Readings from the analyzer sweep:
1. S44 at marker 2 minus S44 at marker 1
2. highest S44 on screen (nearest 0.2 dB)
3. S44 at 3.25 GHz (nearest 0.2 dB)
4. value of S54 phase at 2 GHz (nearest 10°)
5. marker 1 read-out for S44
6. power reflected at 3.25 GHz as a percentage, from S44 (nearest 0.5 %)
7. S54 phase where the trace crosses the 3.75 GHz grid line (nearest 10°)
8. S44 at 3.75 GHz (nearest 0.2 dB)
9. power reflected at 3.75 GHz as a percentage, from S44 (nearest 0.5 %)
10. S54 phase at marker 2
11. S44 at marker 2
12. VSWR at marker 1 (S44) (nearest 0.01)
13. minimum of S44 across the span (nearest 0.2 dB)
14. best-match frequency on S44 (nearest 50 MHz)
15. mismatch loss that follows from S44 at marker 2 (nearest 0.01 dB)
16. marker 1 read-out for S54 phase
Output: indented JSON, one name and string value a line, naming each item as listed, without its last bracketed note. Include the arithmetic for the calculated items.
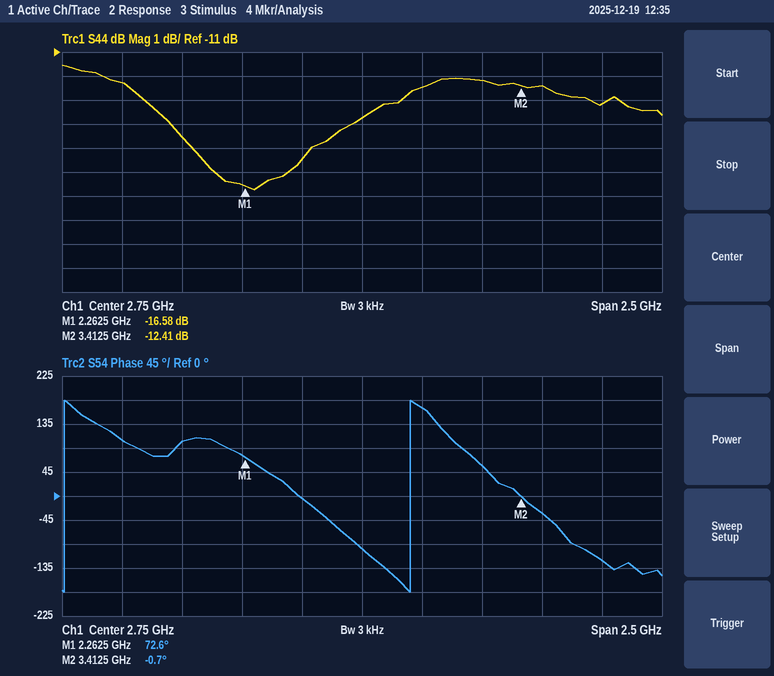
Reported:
{
  "S44 at marker 2 minus S44 at marker 1": "-12.41 − (-16.58) = 4.17 dB",
  "highest S44 on screen": "-11.6 dB",
  "S44 at 3.25 GHz": "-12.2 dB",
  "value of S54 phase at 2 GHz": "100°",
  "marker 1 read-out for S44": "-16.58 dB",
  "power reflected at 3.25 GHz as a percentage, from S44": "10^(-12.2/10) ≈ 6.0 %",
  "S54 phase where the trace crosses the 3.75 GHz grid line": "-120°",
  "S44 at 3.75 GHz": "-13.2 dB",
  "power reflected at 3.75 GHz as a percentage, from S44": "10^(-13.2/10) ≈ 4.79 %, so 5.0 % to the nearest 0.5 %",
  "S54 phase at marker 2": "-0.7°",
  "S44 at marker 2": "-12.41 dB",
  "VSWR at marker 1 (S44)": "(1 + 0.1483)/(1 − 0.1483) ≈ 1.35",
  "minimum of S44 across the span": "-16.8 dB",
  "best-match frequency on S44": "2.30 GHz",
  "mismatch loss that follows from S44 at marker 2": "−10 log10(1 − 10^(-12.41/10)) ≈ 0.26 dB",
  "marker 1 read-out for S54 phase": "72.6°"
}
